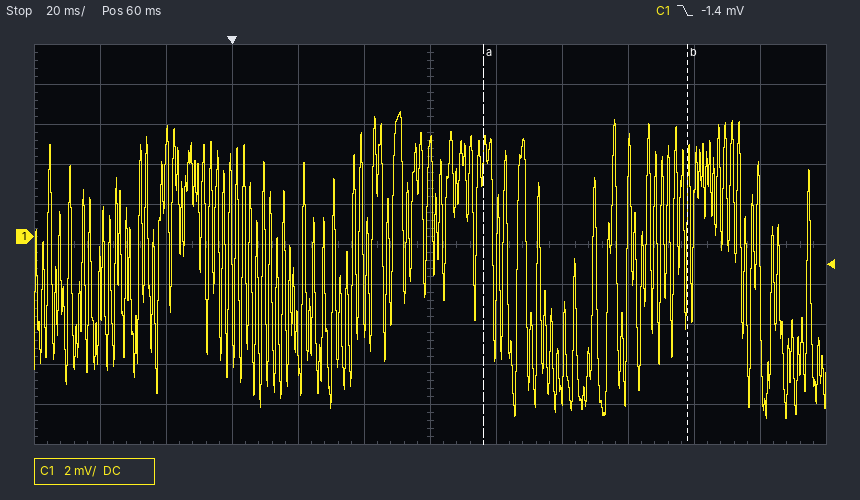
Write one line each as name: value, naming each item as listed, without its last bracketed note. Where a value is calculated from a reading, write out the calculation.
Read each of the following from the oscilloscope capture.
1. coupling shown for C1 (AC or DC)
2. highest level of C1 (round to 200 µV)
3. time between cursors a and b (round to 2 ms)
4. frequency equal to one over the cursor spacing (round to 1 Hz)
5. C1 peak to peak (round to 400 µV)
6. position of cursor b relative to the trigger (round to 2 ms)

coupling shown for C1: DC
highest level of C1: 6.2 mV
time between cursors a and b: 62 ms
frequency equal to one over the cursor spacing: 1 / 62 ms ≈ 16 Hz
C1 peak to peak: 15.2 mV
position of cursor b relative to the trigger: +138 ms
